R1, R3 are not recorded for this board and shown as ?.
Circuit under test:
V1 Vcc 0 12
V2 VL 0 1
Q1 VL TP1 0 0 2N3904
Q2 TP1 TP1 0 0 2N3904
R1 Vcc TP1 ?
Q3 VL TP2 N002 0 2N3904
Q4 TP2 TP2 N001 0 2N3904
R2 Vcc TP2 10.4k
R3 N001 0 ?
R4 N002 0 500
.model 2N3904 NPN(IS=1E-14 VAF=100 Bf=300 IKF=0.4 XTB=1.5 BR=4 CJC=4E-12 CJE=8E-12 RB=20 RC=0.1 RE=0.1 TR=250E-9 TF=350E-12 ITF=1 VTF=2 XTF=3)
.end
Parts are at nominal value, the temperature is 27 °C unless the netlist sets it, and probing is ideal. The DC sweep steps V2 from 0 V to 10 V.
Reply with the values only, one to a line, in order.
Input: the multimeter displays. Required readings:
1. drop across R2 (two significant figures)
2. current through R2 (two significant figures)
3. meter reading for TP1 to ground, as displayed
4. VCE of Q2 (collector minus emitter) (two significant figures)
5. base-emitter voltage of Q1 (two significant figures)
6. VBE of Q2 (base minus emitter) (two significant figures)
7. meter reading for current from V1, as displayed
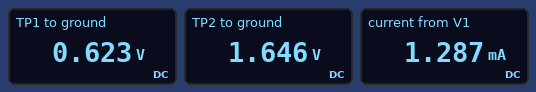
10 V
1.0 mA
0.623 V
620 mV
620 mV
620 mV
1.287 mA
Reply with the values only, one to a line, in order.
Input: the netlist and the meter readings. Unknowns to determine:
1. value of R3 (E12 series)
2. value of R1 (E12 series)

1.2 kΩ
39 kΩ
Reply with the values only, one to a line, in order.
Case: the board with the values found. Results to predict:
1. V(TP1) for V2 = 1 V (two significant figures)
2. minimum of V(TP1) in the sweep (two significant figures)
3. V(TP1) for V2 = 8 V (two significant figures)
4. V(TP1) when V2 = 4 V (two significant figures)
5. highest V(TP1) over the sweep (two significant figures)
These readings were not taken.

620 mV
620 mV
620 mV
620 mV
620 mV
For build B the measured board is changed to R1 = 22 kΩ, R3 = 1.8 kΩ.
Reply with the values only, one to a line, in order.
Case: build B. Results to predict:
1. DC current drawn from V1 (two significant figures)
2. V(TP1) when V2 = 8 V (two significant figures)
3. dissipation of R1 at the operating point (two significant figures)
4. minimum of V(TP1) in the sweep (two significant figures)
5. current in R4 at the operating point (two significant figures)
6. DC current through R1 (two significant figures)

1.5 mA
640 mV
5.9 mW
630 mV
2.0 mA
520 µA
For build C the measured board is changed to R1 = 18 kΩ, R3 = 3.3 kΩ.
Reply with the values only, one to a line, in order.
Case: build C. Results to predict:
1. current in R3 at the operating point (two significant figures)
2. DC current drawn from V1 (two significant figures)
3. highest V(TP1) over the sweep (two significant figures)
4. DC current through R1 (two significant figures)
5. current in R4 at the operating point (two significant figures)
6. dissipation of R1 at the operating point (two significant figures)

320 µA
1.6 mA
640 mV
630 µA
2.0 mA
7.2 mW
